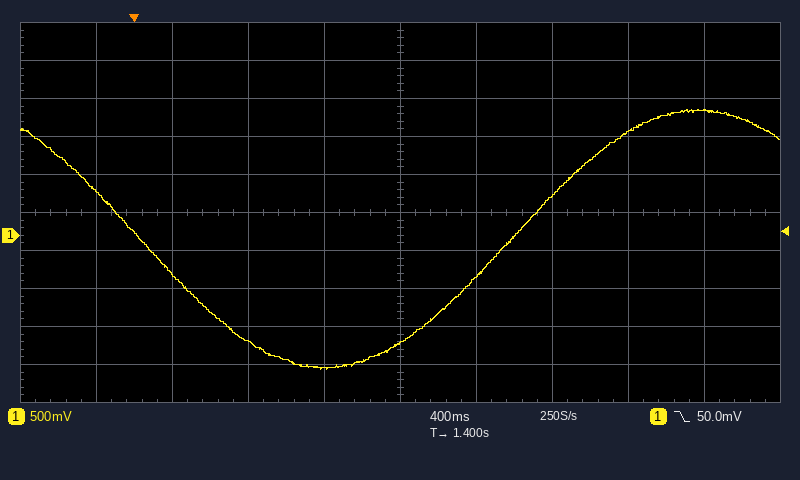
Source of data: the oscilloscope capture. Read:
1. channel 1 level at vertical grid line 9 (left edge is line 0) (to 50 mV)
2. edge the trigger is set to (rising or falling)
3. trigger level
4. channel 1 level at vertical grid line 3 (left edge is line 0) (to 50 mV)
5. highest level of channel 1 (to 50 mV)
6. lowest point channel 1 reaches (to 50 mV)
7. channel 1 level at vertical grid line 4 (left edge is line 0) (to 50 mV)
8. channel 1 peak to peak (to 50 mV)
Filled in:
1.65 V
falling
50.0 mV
-1.40 V
1.65 V
-1.75 V
-1.75 V
3.40 V
